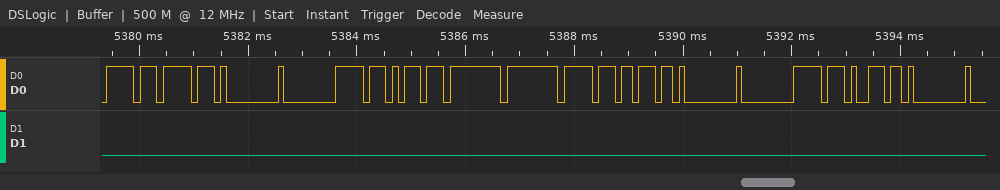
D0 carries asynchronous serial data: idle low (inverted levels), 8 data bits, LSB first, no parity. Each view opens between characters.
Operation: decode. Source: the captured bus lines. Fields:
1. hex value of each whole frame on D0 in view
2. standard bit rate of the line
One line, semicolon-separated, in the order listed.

10, 10, FF, FF, 10, 11, 00, 00, 10, 22, FF, FF, 10, 23, FF; 9600 baud
